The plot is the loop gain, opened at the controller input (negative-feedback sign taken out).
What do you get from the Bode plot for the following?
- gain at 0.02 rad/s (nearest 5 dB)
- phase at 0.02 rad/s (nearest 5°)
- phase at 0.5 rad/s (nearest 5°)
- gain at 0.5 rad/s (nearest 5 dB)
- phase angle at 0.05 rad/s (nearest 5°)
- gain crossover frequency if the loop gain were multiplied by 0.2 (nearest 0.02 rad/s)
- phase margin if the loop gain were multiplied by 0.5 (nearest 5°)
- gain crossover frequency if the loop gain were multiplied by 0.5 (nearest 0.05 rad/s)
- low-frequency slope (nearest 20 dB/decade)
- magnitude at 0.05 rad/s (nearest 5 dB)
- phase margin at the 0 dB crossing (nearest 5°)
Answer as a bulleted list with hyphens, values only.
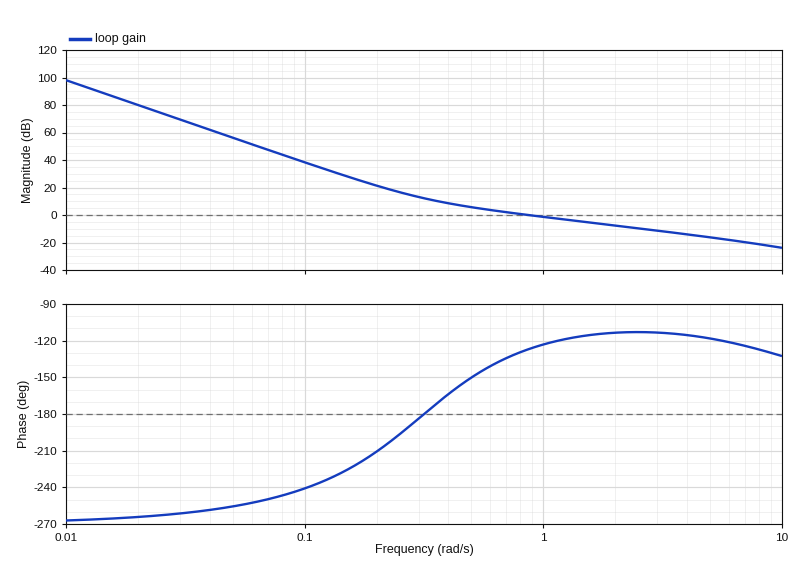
- 80 dB
- -265°
- -150°
- 5 dB
- -255°
- 0.28 rad/s
- 30°
- 0.50 rad/s
- -60 dB/decade
- 55 dB
- 55°
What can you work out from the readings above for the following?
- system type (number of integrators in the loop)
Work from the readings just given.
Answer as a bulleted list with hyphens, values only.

- 3
